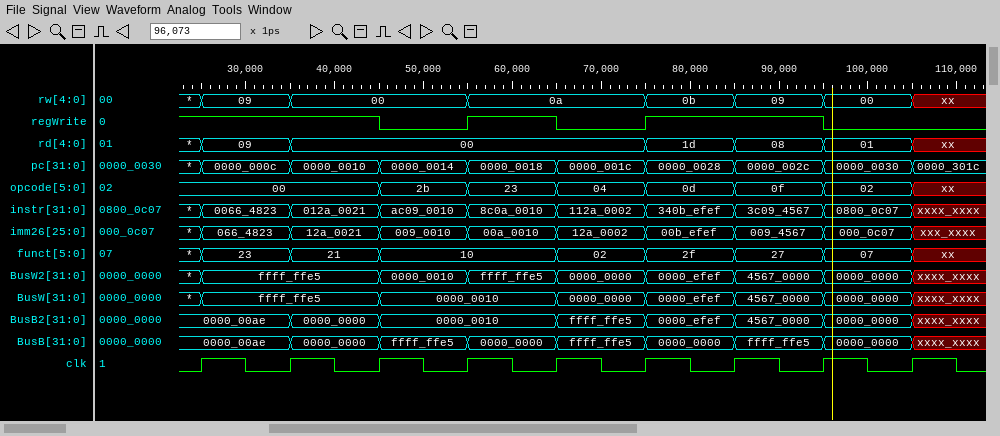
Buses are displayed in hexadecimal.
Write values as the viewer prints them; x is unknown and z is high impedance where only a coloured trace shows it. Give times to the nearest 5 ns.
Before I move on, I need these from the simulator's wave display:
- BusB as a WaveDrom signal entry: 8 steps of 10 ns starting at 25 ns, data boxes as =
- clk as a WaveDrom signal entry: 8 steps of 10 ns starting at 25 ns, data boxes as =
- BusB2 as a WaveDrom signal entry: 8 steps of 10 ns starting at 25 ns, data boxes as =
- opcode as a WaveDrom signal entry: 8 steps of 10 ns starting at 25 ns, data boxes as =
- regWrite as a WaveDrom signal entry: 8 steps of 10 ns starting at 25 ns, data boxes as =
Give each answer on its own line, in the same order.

{name: 'BusB', wave: '========', data: '0000_00ae 0000_0000 ffff_ffe5 0000_0000 ffff_ffe5 0000_0000 ffff_ffe5 0000_0000'}
{name: 'clk', wave: 'p.......'}
{name: 'BusB2', wave: '===.====', data: '0000_00ae 0000_0000 0000_0010 ffff_ffe5 0000_efef 4567_0000 0000_0000'}
{name: 'opcode', wave: '=.======', data: '00 2b 23 04 0d 0f 02'}
{name: 'regWrite', wave: '1.0101.0'}
